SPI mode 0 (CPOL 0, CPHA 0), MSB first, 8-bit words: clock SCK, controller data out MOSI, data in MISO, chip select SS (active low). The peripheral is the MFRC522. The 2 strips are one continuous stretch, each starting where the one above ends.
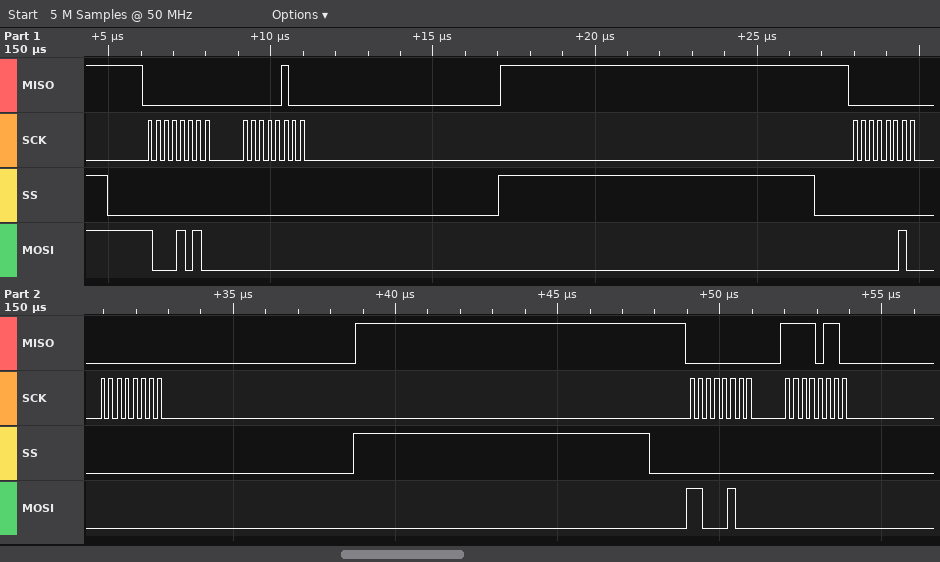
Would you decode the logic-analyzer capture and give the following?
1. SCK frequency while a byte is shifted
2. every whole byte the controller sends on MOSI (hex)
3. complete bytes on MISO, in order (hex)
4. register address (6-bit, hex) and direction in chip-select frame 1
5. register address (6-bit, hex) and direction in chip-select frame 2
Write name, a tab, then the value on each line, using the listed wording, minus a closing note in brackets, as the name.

SCK frequency while a byte is shifted	4 MHz
every whole byte the controller sends on MOSI	0x8A 0x00 0x02 0x00 0xC4 0x00
complete bytes on MISO, in order	0x00 0x04 0x00 0x00 0x00 0xF6
register address (6-bit, hex) and direction in chip-select frame 1	0x05 read
register address (6-bit, hex) and direction in chip-select frame 2	0x01 write
